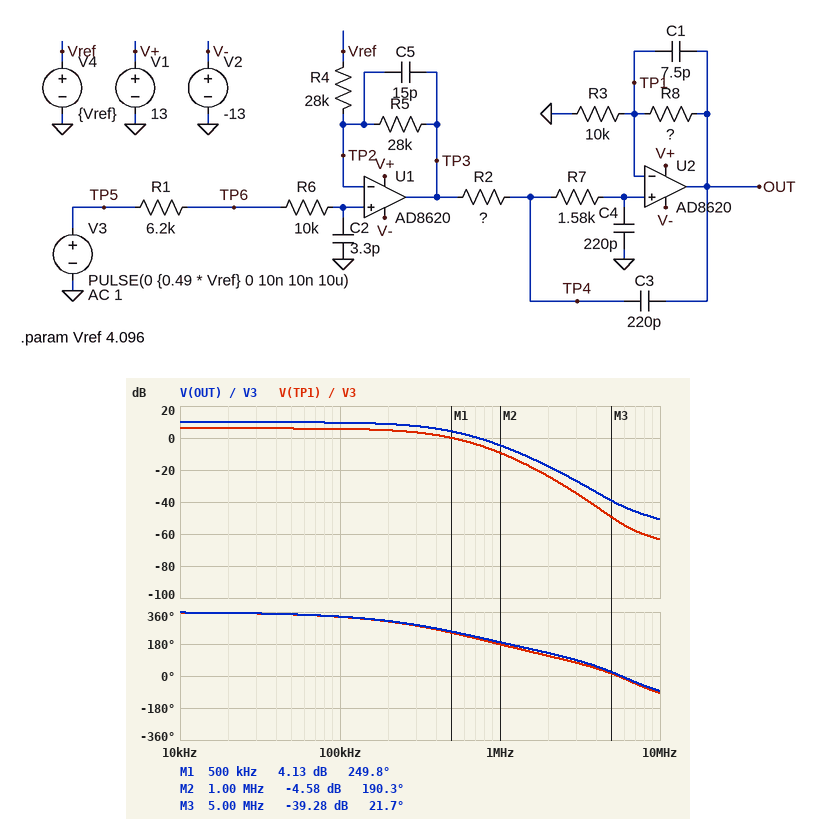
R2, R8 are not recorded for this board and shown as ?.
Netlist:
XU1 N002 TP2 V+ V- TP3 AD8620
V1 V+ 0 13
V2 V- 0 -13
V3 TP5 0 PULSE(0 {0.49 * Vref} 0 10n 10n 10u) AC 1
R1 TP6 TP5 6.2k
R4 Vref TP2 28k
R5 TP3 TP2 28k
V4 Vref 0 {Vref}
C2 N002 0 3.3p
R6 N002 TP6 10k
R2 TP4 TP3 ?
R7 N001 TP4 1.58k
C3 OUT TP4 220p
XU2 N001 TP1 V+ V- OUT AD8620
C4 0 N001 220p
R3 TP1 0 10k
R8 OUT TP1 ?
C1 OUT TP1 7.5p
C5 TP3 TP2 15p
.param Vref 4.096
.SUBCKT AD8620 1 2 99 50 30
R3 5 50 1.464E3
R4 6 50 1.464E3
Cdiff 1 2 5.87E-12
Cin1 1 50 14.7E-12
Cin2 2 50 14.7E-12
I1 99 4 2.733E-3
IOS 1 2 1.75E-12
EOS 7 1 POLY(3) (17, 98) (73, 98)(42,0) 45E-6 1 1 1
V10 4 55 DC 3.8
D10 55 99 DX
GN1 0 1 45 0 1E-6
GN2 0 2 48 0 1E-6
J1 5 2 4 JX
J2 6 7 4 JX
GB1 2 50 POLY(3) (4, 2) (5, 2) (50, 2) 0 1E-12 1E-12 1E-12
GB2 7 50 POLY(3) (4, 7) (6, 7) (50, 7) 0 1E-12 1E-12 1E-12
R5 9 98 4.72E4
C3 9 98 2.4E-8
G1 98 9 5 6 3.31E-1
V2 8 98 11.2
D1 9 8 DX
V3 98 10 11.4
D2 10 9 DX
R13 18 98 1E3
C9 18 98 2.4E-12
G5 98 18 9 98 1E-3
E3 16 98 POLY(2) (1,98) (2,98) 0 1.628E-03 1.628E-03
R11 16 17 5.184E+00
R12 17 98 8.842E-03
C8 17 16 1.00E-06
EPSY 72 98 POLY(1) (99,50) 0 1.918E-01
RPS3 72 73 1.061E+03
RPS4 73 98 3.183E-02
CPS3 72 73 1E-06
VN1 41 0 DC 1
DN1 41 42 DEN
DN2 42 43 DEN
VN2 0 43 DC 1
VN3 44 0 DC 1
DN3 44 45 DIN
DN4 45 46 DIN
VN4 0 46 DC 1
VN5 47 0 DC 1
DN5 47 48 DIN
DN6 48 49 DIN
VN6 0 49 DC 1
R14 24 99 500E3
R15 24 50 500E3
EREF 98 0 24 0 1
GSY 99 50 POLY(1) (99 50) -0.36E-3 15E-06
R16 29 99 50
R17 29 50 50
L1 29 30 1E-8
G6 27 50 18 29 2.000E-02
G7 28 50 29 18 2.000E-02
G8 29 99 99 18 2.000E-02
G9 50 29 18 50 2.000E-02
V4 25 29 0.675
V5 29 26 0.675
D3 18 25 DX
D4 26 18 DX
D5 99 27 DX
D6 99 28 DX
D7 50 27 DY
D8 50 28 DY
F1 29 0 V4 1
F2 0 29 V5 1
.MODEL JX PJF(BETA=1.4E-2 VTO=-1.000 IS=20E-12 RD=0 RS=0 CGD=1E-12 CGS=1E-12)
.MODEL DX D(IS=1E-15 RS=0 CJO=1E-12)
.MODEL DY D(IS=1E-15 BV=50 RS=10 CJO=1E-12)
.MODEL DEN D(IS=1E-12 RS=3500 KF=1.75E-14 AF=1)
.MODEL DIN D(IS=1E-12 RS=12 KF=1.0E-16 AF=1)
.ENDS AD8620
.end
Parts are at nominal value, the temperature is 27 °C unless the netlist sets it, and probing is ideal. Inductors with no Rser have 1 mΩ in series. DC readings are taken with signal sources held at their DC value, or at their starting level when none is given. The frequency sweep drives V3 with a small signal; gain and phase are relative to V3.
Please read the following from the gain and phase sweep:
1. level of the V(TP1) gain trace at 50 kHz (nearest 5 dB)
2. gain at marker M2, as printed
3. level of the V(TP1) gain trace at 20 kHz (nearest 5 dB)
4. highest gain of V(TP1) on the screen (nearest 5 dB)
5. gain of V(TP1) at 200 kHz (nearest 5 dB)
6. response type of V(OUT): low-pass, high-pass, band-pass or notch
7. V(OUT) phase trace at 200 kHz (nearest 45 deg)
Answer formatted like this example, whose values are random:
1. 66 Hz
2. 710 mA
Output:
1. 5 dB
2. -4.58 dB
3. 5 dB
4. 5 dB
5. 5 dB
6. low-pass
7. 315 deg
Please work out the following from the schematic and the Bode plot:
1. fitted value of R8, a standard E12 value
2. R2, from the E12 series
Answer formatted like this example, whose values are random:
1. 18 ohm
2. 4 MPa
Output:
1. 5.6 kΩ
2. 680 Ω
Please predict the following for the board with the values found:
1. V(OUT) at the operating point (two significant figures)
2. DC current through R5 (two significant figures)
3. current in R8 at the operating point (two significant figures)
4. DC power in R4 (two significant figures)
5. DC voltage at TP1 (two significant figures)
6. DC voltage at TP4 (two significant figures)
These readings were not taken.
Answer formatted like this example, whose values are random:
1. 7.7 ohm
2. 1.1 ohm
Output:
1. -6.4 V
2. 150 µA
3. 410 µA
4. 600 µW
5. -4.1 V
6. -4.1 V
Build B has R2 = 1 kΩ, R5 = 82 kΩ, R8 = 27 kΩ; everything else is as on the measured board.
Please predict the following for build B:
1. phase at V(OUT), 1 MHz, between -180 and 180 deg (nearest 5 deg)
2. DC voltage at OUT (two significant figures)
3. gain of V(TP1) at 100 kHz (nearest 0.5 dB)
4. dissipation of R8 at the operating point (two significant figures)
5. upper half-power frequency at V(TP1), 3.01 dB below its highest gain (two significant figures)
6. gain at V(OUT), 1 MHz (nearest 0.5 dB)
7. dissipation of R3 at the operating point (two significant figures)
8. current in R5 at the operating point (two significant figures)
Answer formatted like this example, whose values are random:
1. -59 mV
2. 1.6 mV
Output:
1. -30 deg
2. -12 V
3. -29.0 dB
4. 3.0 mW
5. 690 kHz
6. -36.0 dB
7. 1.1 mW
8. 150 µA
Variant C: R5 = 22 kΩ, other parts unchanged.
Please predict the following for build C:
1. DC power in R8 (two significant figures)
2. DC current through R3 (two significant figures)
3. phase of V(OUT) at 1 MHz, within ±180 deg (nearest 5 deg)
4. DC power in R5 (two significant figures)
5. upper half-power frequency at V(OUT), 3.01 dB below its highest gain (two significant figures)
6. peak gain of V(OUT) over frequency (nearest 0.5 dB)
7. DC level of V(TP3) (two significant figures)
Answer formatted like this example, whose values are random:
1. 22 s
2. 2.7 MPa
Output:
1. 580 µW
2. 320 µA
3. -165 deg
4. 470 µW
5. 360 kHz
6. 9.0 dB
7. -3.2 V
